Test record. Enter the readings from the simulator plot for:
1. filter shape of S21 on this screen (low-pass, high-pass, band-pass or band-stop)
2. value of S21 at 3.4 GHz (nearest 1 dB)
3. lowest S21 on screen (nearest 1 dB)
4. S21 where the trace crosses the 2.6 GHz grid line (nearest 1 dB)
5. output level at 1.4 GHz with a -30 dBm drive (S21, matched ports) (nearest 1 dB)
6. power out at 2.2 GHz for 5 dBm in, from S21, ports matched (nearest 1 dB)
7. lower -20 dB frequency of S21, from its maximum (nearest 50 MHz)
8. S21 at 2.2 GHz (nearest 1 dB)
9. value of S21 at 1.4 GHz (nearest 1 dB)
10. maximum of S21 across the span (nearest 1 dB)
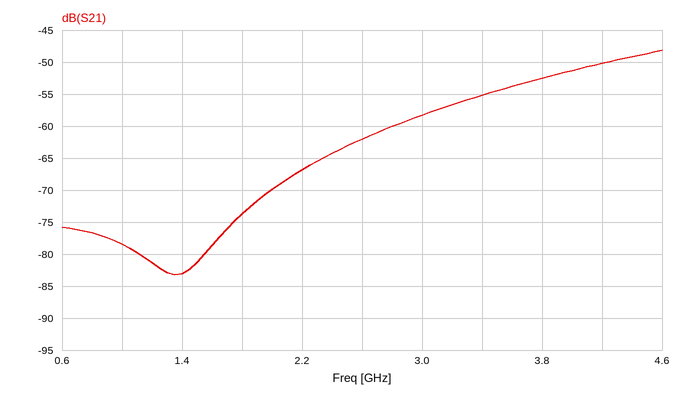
high-pass
-55 dB
-83 dB
-62 dB
-113 dBm
-62 dBm
2.10 GHz
-67 dB
-83 dB
-48 dB
